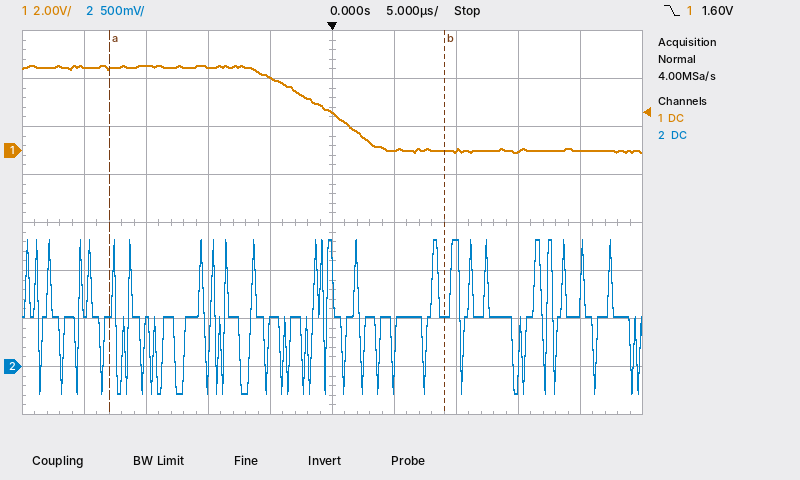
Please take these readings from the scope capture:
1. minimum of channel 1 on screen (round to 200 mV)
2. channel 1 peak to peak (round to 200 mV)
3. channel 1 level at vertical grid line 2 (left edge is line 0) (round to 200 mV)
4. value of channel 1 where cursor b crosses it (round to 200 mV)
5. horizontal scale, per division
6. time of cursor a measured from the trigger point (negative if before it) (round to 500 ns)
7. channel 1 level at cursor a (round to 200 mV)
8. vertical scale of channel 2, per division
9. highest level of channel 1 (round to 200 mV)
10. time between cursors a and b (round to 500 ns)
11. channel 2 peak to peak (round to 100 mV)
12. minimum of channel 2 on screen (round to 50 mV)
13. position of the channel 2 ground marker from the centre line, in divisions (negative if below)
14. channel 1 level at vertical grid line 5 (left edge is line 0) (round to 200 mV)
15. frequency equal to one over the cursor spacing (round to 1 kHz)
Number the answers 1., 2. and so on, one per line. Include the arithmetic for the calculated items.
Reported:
1. 0.0 V
2. 3.6 V − (0.0 V) = 3.6 V
3. 3.6 V
4. 0.0 V
5. 5 µs
6. -18.0 µs
7. 3.4 V
8. 500 mV
9. 3.6 V
10. 27.0 µs
11. 1.60 V
12. -300 mV
13. -3.0 div
14. 1.6 V
15. 1 / 27.0 µs ≈ 37 kHz
